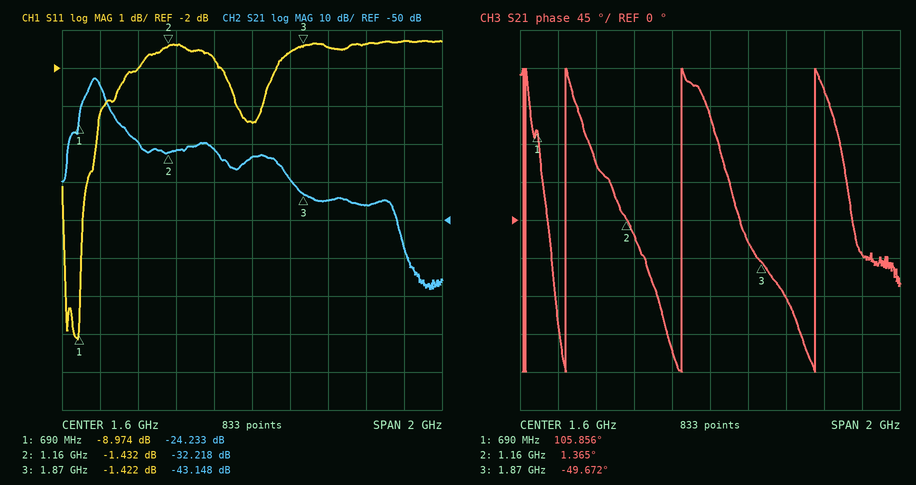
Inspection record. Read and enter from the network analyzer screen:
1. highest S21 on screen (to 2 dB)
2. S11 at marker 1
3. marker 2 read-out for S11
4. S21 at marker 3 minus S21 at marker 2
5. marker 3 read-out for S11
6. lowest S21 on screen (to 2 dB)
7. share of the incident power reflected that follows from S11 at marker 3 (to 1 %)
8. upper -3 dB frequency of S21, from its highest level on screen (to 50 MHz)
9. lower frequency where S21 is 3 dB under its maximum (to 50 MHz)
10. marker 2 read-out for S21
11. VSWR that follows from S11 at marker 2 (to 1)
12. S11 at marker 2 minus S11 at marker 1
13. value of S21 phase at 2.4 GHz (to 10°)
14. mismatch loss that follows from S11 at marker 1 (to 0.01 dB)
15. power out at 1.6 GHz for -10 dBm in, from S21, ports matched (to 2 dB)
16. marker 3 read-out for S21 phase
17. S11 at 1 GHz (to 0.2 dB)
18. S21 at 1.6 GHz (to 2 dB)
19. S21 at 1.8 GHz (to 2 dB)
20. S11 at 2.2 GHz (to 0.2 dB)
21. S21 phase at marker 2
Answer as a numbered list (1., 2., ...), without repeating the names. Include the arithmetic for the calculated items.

1. -12 dB
2. -8.974 dB
3. -1.432 dB
4. -43.148 − (-32.218) = -10.930 dB
5. -1.422 dB
6. -68 dB
7. 10^(-1.422/10) ≈ 72 %
8. 800 MHz
9. 750 MHz
10. -32.218 dB
11. (1 + 0.8480)/(1 − 0.8480) ≈ 12
12. -1.432 − (-8.974) = 7.542 dB
13. -40°
14. −10 log10(1 − 10^(-8.974/10)) ≈ 0.59 dB
15. -10 dBm + (-34 dB) = -44 dBm
16. -49.672°
17. -2.0 dB
18. -34 dB
19. -40 dB
20. -1.4 dB
21. 1.365°
